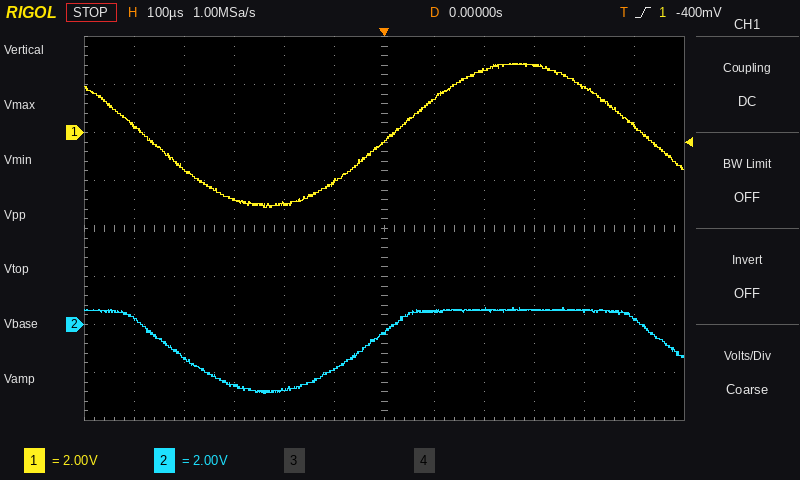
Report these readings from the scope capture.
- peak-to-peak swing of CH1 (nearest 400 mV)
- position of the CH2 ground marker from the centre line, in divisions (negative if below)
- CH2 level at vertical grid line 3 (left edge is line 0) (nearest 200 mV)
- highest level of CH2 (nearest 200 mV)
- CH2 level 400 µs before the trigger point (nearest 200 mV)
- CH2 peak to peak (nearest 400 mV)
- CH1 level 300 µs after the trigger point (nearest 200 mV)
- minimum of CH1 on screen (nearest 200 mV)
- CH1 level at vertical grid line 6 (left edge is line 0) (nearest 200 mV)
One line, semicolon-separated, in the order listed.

6.0 V; -2.0 div; -2.6 V; 800 mV; -1.4 V; 3.6 V; 2.8 V; -3.2 V; -400 mV
